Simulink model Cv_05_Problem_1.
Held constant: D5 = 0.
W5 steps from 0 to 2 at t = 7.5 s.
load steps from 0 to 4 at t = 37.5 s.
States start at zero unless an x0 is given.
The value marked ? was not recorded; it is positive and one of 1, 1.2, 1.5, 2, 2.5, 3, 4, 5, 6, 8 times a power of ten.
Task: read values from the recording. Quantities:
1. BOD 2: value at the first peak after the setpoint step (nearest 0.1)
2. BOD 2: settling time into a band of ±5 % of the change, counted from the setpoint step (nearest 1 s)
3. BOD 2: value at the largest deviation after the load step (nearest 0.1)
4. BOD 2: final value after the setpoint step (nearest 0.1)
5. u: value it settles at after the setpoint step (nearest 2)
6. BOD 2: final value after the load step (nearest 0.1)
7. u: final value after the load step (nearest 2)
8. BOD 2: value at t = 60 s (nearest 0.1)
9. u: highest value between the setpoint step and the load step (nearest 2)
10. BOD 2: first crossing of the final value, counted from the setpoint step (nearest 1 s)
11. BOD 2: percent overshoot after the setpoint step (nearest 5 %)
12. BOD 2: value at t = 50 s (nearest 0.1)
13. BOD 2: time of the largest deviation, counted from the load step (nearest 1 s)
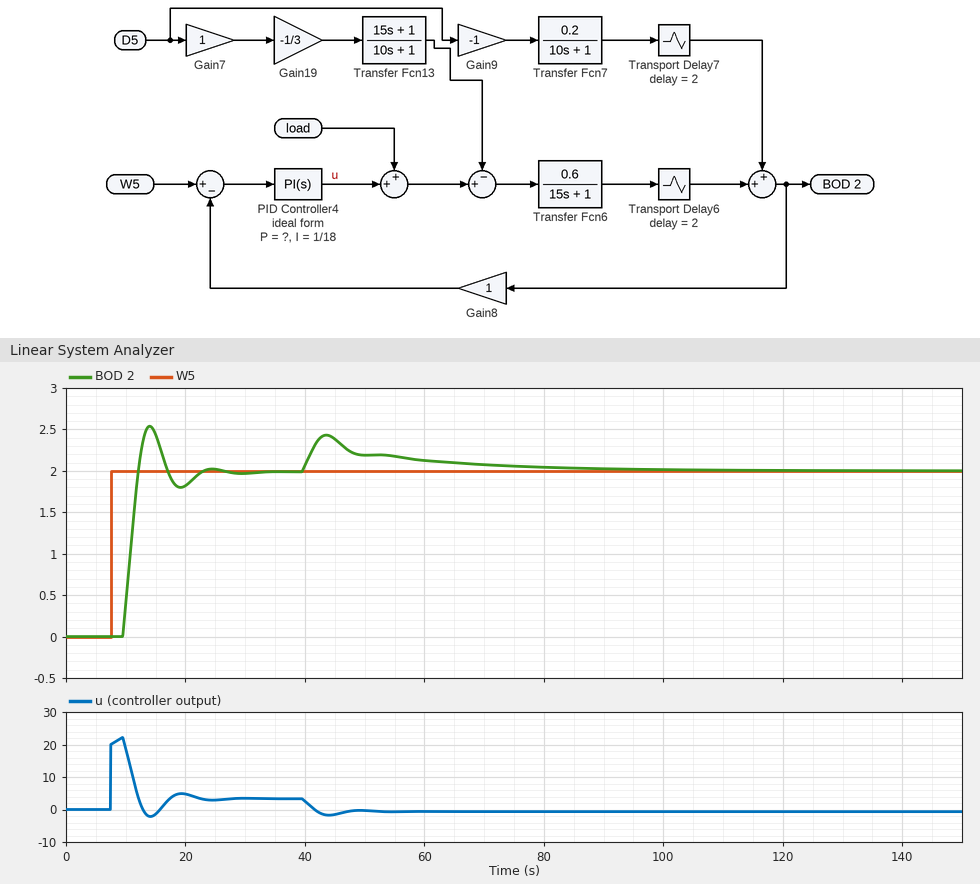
2.5
14 s
2.4
2.0
4
2.0
0
2.1
22
5 s
25 %
2.2
6 s
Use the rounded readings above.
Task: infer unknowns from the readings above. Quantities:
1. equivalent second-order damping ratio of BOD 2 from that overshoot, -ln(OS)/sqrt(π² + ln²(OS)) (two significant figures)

0.40
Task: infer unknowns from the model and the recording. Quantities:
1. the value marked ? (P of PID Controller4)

10
